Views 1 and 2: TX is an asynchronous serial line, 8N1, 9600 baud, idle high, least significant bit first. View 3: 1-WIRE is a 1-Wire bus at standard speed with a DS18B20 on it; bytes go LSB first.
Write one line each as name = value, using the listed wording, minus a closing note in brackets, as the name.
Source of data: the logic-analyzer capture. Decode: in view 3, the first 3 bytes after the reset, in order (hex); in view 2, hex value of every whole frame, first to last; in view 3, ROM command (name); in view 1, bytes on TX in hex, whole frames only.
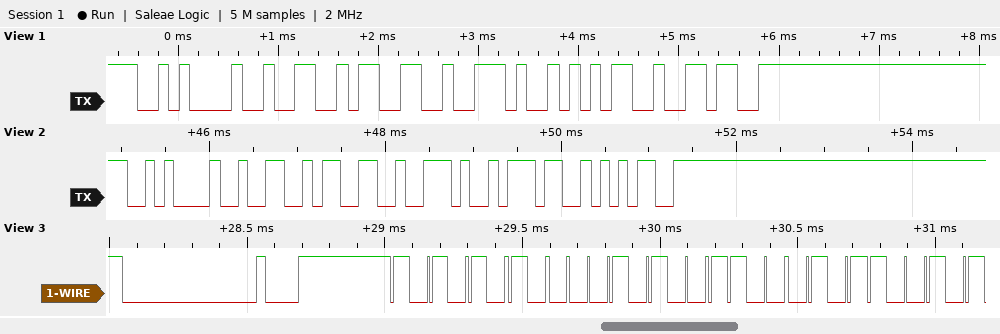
in view 3, the first 3 bytes after the reset, in order = 55 28 A3
in view 2, hex value of every whole frame, first to last = 0x0A 0x32 0x33 0x2E 0x37 0x35
in view 3, ROM command = Match ROM
in view 1, bytes on TX in hex, whole frames only = 0x0A 0x32 0x33 0x2E 0x35 0x36
